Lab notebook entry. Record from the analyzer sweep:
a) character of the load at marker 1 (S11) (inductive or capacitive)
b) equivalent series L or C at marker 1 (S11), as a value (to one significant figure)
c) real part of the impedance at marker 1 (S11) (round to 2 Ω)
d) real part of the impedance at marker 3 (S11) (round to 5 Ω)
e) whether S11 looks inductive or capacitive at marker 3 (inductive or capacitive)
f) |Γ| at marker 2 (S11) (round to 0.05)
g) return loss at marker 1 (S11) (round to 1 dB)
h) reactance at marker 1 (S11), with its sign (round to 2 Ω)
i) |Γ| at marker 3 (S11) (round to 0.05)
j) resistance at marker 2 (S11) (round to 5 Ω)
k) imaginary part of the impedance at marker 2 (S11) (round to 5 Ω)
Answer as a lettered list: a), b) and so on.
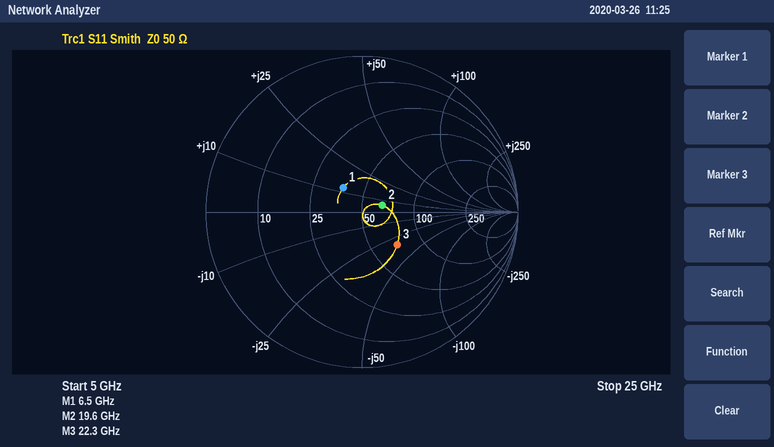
a) inductive
b) 300 pH
c) 38 Ω
d) 70 Ω
e) capacitive
f) 0.15
g) 14 dB
h) +12 Ω
i) 0.30
j) 65 Ω
k) +5 Ω
